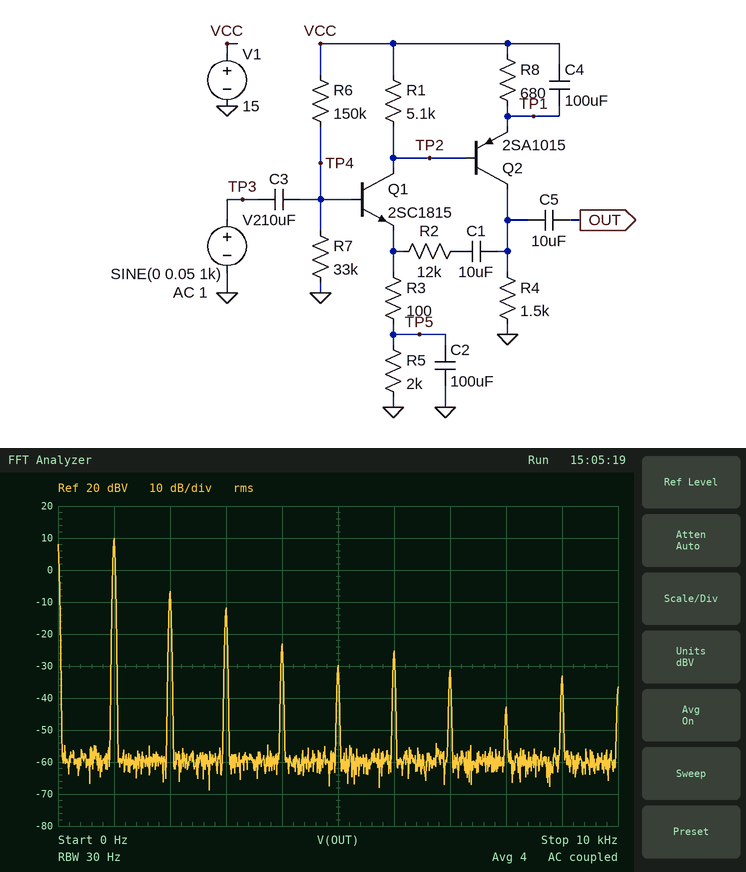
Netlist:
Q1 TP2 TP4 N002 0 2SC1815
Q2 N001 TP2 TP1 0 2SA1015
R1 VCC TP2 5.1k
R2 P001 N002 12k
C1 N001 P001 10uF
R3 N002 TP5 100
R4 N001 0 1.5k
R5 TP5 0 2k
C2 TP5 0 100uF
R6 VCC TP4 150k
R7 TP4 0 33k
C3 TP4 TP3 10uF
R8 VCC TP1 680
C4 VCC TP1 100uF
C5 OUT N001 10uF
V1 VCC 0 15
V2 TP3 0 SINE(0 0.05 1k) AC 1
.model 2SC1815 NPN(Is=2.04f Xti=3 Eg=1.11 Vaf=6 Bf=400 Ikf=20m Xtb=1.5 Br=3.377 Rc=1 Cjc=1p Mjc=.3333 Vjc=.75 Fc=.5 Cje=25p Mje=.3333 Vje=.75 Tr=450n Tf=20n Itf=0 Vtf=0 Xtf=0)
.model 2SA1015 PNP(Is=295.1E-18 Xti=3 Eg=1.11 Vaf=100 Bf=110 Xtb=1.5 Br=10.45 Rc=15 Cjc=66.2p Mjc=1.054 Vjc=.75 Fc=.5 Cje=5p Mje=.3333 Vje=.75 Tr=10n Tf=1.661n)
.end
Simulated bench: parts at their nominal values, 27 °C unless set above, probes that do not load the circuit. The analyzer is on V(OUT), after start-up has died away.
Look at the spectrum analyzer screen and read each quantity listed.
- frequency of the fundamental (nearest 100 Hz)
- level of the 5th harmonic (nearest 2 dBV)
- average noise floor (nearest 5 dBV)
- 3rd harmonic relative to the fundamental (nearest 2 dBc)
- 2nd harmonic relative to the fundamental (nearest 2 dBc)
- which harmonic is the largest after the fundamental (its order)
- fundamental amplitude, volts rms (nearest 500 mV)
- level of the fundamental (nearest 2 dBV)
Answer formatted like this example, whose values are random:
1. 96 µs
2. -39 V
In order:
1. 1.0 kHz
2. -30 dBV
3. -60 dBV
4. -22 dBc
5. -16 dBc
6. 2
7. 3.0 V
8. 10 dBV
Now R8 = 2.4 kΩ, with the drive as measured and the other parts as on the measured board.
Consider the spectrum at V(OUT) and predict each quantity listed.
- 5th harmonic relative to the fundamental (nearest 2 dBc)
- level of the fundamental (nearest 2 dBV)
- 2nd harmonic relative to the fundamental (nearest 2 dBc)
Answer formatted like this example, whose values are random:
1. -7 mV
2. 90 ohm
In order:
1. -30 dBc
2. 8 dBV
3. -10 dBc
